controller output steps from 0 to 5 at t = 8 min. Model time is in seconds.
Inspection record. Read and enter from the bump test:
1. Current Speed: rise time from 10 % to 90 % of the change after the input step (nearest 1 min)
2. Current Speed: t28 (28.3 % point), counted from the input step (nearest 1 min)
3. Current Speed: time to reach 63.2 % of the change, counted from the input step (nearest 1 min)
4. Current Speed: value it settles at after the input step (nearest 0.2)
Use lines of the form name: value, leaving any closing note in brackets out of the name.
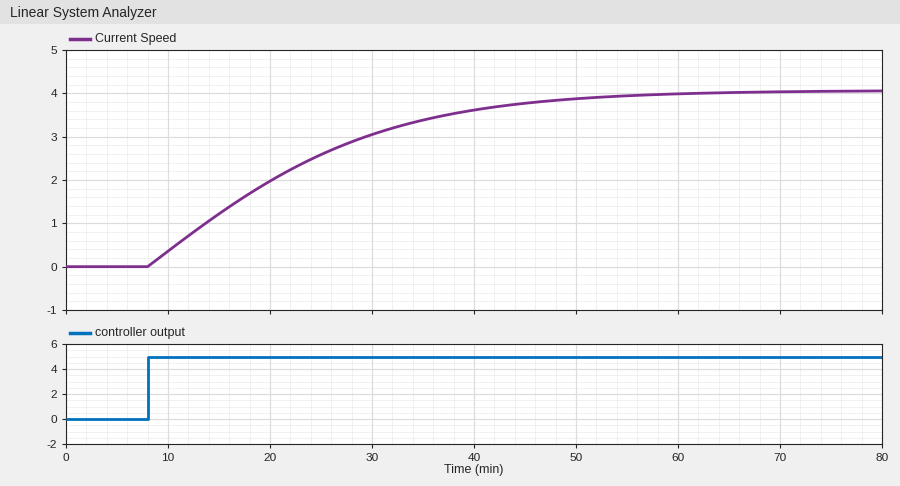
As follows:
Current Speed: rise time from 10 % to 90 % of the change after the input step: 31 min
Current Speed: t28 (28.3 % point), counted from the input step: 7 min
Current Speed: time to reach 63.2 % of the change, counted from the input step: 17 min
Current Speed: value it settles at after the input step: 4.0
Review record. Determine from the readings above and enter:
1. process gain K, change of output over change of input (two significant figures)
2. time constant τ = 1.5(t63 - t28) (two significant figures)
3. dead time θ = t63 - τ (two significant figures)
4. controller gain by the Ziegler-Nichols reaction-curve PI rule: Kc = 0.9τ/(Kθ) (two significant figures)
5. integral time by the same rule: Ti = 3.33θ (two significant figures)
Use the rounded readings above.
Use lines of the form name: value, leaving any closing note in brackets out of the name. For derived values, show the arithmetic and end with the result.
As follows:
process gain K, change of output over change of input: (4 - 0) / 5 = 0.80
time constant τ = 1.5(t63 - t28): 1.5 × (17 - 7) = 15 min
dead time θ = t63 - τ: 17 - 15 = 2.0 min
controller gain by the Ziegler-Nichols reaction-curve PI rule: Kc = 0.9τ/(Kθ): 0.9 × 15 / (0.8 × 2) = 8.4
integral time by the same rule: Ti = 3.33θ: 3.33 × 2 = 6.7 min
